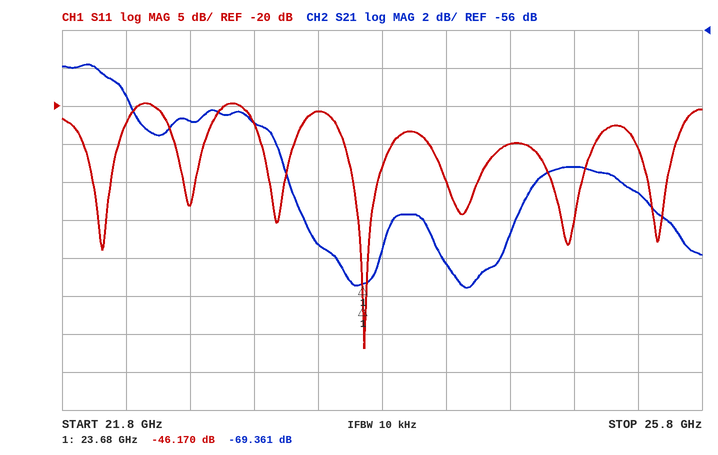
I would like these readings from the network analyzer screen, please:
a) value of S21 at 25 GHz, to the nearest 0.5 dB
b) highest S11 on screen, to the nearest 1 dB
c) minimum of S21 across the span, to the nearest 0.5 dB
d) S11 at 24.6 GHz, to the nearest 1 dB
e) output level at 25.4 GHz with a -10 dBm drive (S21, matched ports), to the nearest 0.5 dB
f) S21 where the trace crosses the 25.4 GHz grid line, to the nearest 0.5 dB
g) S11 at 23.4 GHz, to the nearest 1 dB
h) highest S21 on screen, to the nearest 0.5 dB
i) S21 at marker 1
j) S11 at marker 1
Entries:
-63.0 dB
-20 dB
-69.5 dB
-25 dB
-74.5 dBm
-64.5 dB
-21 dB
-58.0 dB
-69.361 dB
-46.170 dB
